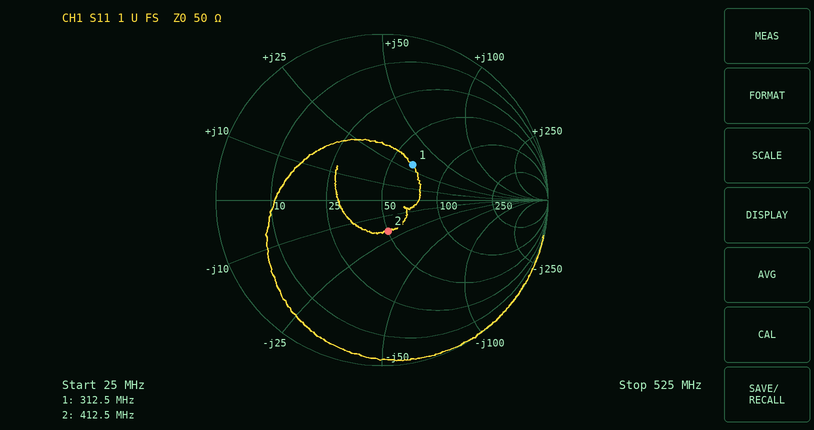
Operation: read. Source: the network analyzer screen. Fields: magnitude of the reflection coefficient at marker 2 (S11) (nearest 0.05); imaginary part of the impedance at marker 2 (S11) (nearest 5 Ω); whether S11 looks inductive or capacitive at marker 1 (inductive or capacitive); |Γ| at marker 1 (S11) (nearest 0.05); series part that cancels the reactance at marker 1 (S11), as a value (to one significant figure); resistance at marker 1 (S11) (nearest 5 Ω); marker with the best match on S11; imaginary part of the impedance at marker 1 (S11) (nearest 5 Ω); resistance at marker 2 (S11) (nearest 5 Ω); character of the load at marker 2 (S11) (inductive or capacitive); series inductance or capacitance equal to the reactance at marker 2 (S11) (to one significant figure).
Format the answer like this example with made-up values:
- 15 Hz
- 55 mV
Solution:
- 0.20
- -20 Ω
- inductive
- 0.30
- 20 pF
- 65 Ω
- marker 2
- +30 Ω
- 50 Ω
- capacitive
- 20 pF
